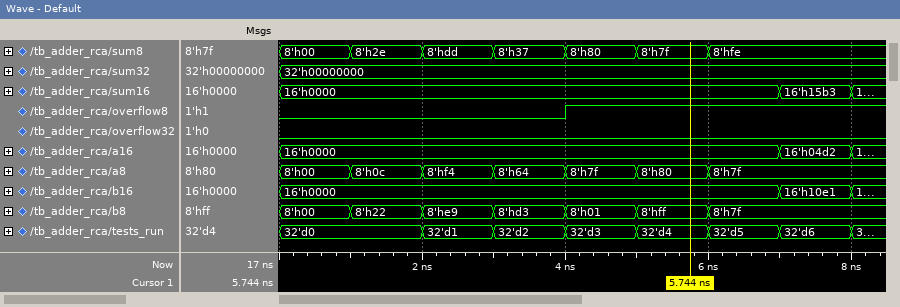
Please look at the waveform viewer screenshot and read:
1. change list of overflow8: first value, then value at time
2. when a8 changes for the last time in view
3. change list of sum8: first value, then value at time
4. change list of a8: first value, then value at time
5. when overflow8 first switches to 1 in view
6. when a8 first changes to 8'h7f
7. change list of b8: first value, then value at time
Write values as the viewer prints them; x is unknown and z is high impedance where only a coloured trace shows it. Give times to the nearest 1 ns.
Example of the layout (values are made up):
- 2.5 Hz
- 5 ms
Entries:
- 0, 1 at 4 ns
- 6 ns
- 8'h00, 8'h2e at 1 ns, 8'hdd at 2 ns, 8'h37 at 3 ns, 8'h80 at 4 ns, 8'h7f at 5 ns, 8'hfe at 6 ns
- 8'h00, 8'h0c at 1 ns, 8'hf4 at 2 ns, 8'h64 at 3 ns, 8'h7f at 4 ns, 8'h80 at 5 ns, 8'h7f at 6 ns
- 4 ns
- 4 ns
- 8'h00, 8'h22 at 1 ns, 8'he9 at 2 ns, 8'hd3 at 3 ns, 8'h01 at 4 ns, 8'hff at 5 ns, 8'h7f at 6 ns
